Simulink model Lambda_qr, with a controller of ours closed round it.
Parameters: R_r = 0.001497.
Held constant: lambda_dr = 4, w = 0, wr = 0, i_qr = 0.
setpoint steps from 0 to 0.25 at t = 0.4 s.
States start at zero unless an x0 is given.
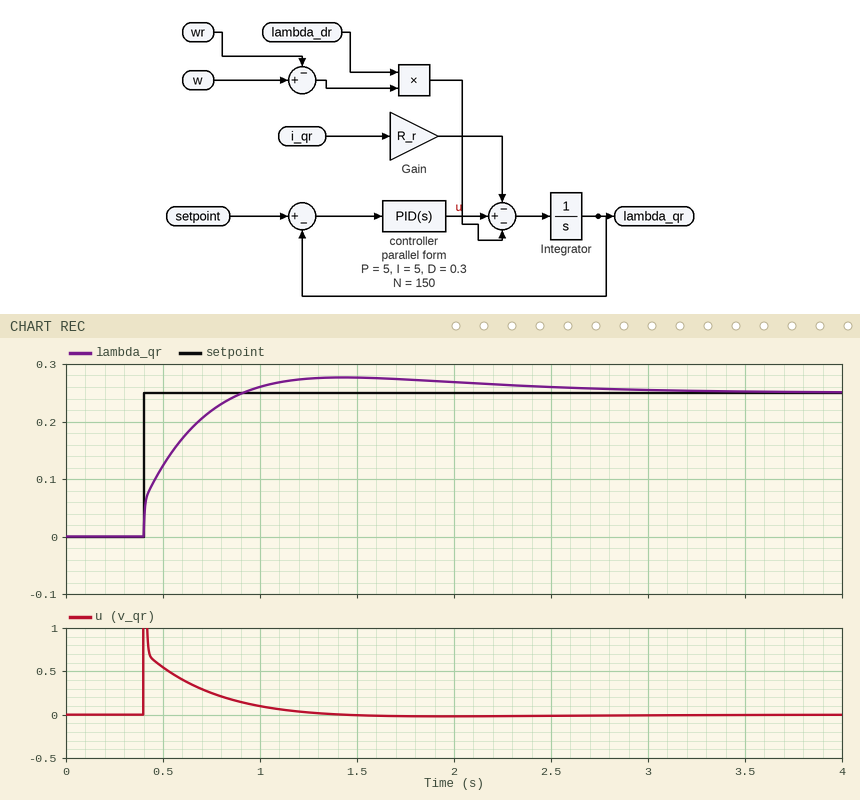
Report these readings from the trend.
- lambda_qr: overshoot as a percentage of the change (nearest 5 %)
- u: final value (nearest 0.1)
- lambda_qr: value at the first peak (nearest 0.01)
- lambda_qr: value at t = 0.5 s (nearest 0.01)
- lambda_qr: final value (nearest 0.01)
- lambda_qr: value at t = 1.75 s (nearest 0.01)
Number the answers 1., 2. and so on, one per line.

1. 10 %
2. 0.0
3. 0.28
4. 0.12
5. 0.25
6. 0.27
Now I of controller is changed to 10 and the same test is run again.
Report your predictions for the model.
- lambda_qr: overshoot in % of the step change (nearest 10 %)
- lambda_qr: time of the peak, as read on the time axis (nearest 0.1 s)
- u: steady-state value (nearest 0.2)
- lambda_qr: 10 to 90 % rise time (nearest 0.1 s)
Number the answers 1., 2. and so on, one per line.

1. 20 %
2. 1.2 s
3. 0.0
4. 0.3 s
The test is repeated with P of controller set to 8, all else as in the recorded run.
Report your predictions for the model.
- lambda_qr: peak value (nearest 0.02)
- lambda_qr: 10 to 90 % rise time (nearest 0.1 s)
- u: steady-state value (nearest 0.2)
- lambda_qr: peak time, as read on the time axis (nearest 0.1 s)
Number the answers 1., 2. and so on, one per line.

1. 0.26
2. 0.3 s
3. 0.0
4. 1.3 s
